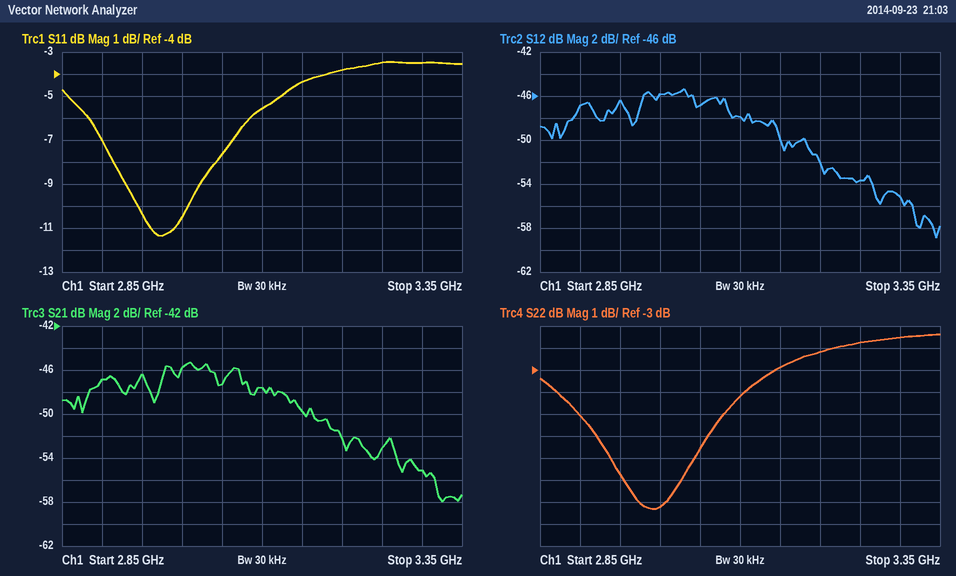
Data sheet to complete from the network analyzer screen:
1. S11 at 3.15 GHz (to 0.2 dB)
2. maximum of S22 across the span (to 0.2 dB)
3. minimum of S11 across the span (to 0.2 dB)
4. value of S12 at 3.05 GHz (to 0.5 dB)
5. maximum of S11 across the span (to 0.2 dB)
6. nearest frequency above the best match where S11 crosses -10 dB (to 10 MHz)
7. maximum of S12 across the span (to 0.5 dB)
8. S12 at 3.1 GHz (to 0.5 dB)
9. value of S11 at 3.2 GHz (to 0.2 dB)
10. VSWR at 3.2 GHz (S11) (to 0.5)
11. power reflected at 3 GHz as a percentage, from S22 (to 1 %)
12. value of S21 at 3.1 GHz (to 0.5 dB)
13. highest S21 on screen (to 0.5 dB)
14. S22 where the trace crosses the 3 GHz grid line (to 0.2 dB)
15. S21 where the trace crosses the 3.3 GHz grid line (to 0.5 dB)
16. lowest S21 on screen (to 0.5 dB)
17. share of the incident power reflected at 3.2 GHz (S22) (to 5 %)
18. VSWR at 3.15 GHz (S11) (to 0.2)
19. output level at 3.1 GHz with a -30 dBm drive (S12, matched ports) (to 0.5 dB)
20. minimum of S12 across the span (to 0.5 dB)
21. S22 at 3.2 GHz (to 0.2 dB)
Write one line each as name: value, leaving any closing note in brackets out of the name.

S11 at 3.15 GHz: -4.4 dB
maximum of S22 across the span: -1.4 dB
minimum of S11 across the span: -11.4 dB
value of S12 at 3.05 GHz: -47.0 dB
maximum of S11 across the span: -3.4 dB
nearest frequency above the best match where S11 crosses -10 dB: 3.01 GHz
maximum of S12 across the span: -45.5 dB
S12 at 3.1 GHz: -48.0 dB
value of S11 at 3.2 GHz: -3.8 dB
VSWR at 3.2 GHz (S11): 4.5
power reflected at 3 GHz as a percentage, from S22: 12 %
value of S21 at 3.1 GHz: -47.5 dB
highest S21 on screen: -45.5 dB
S22 where the trace crosses the 3 GHz grid line: -9.2 dB
S21 where the trace crosses the 3.3 GHz grid line: -55.0 dB
lowest S21 on screen: -58.0 dB
share of the incident power reflected at 3.2 GHz (S22): 60 %
VSWR at 3.15 GHz (S11): 4.0
output level at 3.1 GHz with a -30 dBm drive (S12, matched ports): -78.0 dBm
minimum of S12 across the span: -59.0 dB
S22 at 3.2 GHz: -2.2 dB
